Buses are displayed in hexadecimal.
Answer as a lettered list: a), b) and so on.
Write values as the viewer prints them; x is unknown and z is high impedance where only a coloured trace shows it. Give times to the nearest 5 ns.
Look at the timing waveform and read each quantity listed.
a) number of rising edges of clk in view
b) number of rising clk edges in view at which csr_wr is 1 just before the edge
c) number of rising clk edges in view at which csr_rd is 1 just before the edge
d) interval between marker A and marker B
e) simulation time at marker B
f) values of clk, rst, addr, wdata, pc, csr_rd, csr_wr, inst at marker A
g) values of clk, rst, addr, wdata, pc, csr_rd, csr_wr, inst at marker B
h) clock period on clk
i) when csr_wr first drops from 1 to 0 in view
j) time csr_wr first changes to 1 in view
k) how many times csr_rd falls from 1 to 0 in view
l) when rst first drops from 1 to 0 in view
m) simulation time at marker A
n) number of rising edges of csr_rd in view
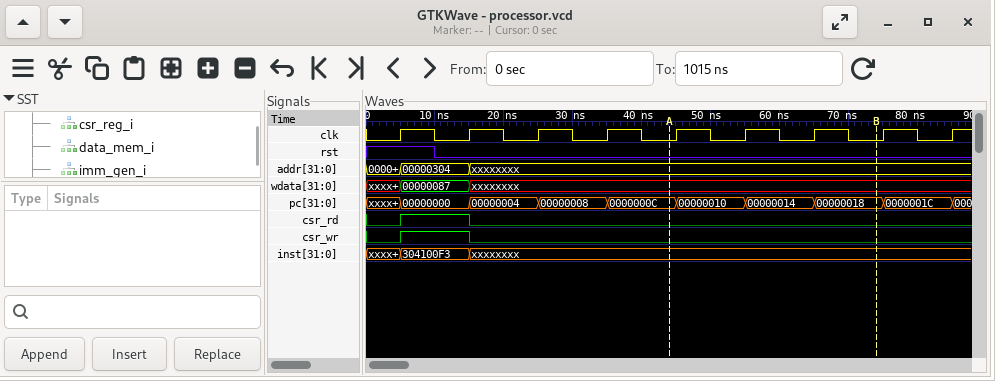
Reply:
a) 9
b) 1
c) 1
d) 30 ns
e) 75 ns
f) clk=0, rst=0, addr=xxxxxxxx, wdata=xxxxxxxx, pc=0000000C, csr_rd=0, csr_wr=0, inst=xxxxxxxx
g) clk=0, rst=0, addr=xxxxxxxx, wdata=xxxxxxxx, pc=00000018, csr_rd=0, csr_wr=0, inst=xxxxxxxx
h) 10 ns
i) 15 ns
j) 5 ns
k) 1
l) 10 ns
m) 45 ns
n) 1
